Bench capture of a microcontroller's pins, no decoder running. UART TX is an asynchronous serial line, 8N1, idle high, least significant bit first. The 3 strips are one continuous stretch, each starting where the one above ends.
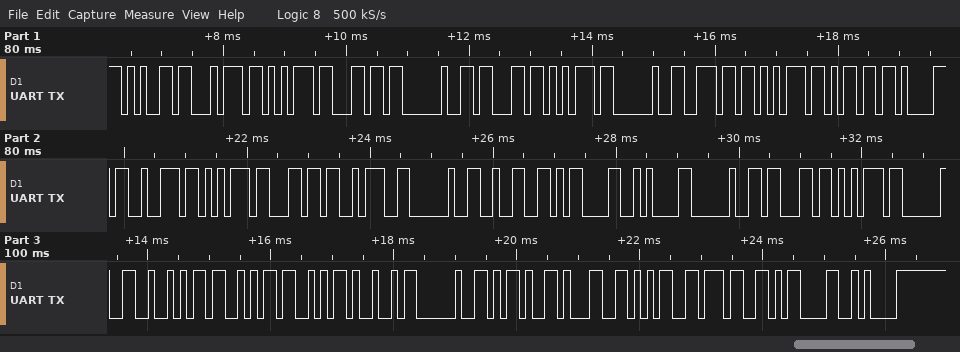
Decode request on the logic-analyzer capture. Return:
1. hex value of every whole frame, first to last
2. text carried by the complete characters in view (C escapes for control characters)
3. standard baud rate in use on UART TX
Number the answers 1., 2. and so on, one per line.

1. 65 74 75 6C 20 63 75 20 6E 75 6D 61 72 75 6C 3A 20 32 0D 0A 20 63 75 20 52 53 53 49 20 2D 31 35 37 0D 0A
2. "etul cu numarul: 2\r\n cu RSSI -157\r\n"
3. 9600 baud
